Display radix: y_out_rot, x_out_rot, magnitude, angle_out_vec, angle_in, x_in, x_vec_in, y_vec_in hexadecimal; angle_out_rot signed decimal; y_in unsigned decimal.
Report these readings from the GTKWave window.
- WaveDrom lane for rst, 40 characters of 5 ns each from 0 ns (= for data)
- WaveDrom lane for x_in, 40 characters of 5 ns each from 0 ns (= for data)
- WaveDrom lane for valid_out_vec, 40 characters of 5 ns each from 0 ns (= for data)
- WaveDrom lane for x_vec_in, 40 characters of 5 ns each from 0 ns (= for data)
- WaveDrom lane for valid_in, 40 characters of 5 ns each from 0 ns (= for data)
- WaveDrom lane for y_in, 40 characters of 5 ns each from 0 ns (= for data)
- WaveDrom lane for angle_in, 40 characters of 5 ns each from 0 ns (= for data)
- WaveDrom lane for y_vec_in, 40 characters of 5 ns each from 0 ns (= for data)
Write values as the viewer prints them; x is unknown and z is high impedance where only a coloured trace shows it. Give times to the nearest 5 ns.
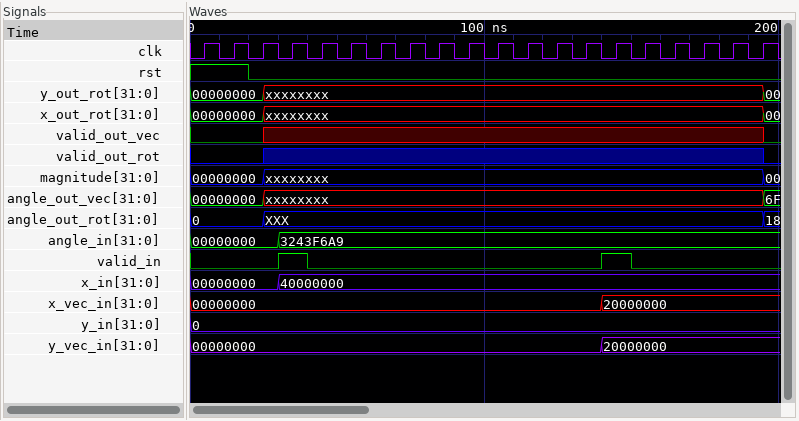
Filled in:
{name: 'rst', wave: '1...0...................................'}
{name: 'x_in', wave: '=.....=.................................', data: '00000000 40000000'}
{name: 'valid_out_vec', wave: '0....x.................................0'}
{name: 'x_vec_in', wave: '=...........................=...........', data: '00000000 20000000'}
{name: 'valid_in', wave: '0.....1.0...................1.0.........'}
{name: 'y_in', wave: '=.......................................', data: '0'}
{name: 'angle_in', wave: '=.....=.................................', data: '00000000 3243F6A9'}
{name: 'y_vec_in', wave: '=...........................=...........', data: '00000000 20000000'}
